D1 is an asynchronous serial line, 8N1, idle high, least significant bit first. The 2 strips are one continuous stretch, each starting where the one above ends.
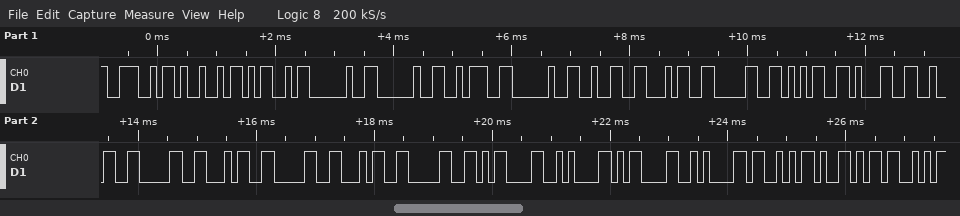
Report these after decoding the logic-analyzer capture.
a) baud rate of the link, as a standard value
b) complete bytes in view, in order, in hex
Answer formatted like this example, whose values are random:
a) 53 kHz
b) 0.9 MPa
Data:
a) 9600 baud
b) 4E 49 4D 20 20 3A 20 32 34 30 35 31 32 30 34 30 34 30 0D 0A 0D 0A 53 59 53
